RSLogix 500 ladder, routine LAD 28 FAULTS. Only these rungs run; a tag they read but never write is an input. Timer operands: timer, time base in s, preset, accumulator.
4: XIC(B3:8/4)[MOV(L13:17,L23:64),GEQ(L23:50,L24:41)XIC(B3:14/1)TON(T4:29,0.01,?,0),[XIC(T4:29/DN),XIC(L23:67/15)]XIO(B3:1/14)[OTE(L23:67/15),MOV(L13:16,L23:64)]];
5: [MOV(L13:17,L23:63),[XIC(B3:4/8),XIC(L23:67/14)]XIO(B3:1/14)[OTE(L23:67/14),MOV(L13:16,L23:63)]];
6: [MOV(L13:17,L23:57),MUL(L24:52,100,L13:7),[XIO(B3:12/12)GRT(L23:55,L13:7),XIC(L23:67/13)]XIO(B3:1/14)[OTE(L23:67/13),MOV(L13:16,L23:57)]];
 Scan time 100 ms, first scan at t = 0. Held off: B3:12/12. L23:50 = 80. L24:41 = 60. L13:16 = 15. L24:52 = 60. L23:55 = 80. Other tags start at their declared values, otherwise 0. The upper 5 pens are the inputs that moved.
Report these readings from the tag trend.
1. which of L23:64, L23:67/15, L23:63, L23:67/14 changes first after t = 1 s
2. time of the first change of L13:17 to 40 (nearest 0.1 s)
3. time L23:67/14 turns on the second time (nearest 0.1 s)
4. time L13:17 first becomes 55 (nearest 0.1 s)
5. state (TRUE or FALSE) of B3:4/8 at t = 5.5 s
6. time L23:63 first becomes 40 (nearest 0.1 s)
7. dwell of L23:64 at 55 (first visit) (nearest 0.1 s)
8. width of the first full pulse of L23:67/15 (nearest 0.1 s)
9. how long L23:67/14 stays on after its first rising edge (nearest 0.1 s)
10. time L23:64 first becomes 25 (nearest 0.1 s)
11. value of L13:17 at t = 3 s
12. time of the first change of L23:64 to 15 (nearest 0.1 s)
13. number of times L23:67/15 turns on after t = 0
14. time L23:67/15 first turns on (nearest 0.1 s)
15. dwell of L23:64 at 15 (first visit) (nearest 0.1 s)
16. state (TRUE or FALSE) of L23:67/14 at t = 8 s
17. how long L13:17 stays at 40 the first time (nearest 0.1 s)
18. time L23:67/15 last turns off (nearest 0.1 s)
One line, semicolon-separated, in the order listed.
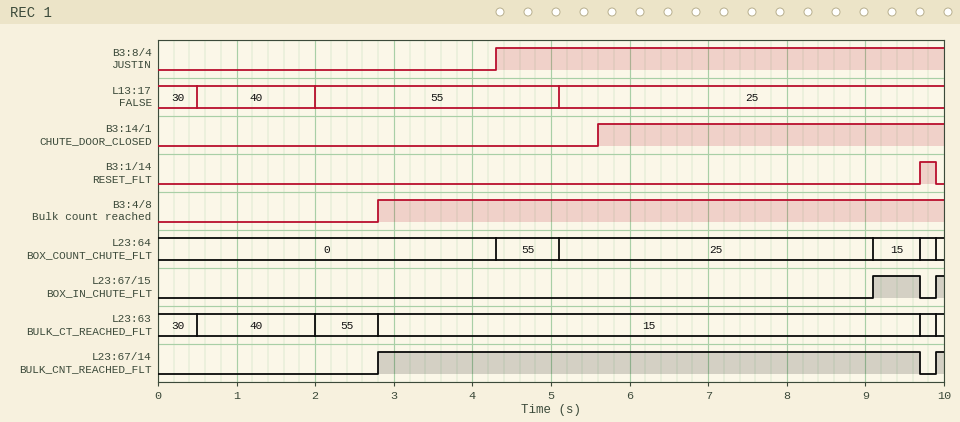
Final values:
L23:63; 0.5 s; 9.9 s; 2.0 s; TRUE; 0.5 s; 0.8 s; 0.6 s; 6.9 s; 5.1 s; 55; 9.1 s; 2; 9.1 s; 0.6 s; TRUE; 1.5 s; 9.7 s
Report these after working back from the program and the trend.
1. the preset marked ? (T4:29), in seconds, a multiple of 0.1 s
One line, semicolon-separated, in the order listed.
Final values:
3.5 s
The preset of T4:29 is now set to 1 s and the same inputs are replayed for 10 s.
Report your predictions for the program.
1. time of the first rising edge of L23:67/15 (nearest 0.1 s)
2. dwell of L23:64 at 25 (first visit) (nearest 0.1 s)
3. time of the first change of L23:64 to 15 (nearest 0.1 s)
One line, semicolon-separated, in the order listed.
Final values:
6.6 s; 1.5 s; 6.6 s
